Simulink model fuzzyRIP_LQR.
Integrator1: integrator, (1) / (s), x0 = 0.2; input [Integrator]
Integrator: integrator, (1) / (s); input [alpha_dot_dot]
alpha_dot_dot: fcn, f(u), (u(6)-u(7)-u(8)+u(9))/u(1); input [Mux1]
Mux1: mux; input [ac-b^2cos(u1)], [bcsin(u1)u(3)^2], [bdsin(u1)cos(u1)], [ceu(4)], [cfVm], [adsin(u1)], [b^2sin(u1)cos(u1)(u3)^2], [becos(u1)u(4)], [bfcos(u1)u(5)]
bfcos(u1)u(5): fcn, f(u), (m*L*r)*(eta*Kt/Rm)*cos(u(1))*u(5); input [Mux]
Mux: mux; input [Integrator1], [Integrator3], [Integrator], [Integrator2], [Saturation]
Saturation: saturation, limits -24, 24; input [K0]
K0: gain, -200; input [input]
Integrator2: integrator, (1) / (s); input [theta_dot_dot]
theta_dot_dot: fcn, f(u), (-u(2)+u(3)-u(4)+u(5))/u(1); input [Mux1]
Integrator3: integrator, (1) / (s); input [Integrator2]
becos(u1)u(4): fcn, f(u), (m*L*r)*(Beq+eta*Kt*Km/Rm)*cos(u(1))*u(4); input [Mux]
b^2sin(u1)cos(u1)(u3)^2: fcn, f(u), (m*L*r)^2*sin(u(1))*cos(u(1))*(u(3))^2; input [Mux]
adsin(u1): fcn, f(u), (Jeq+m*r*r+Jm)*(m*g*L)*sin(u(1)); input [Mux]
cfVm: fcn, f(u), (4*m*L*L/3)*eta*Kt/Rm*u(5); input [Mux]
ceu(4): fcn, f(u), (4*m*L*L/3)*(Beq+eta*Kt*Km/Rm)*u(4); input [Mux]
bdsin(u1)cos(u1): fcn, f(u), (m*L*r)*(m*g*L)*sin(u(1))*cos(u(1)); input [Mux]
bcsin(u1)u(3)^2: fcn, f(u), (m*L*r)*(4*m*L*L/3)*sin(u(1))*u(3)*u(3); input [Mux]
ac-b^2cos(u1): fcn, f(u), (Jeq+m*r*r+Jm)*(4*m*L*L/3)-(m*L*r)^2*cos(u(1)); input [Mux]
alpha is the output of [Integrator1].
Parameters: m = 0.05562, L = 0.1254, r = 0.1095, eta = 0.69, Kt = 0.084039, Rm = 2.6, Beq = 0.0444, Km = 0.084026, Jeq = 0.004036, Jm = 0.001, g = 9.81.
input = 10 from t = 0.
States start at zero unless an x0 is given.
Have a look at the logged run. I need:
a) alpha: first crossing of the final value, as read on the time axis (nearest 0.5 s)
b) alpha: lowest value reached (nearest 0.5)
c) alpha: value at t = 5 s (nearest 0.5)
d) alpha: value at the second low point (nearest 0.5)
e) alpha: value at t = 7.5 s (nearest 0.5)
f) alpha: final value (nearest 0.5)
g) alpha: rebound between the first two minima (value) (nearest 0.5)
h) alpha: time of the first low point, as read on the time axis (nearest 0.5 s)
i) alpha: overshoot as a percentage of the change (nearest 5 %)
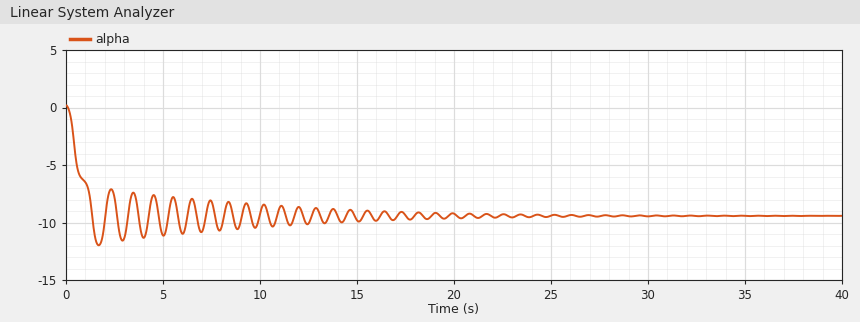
1.5 s
-12.0
-11.0
-11.5
-8.0
-9.5
-7.0
1.5 s
25 %
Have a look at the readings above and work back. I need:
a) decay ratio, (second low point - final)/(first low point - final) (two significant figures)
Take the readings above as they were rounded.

0.80
